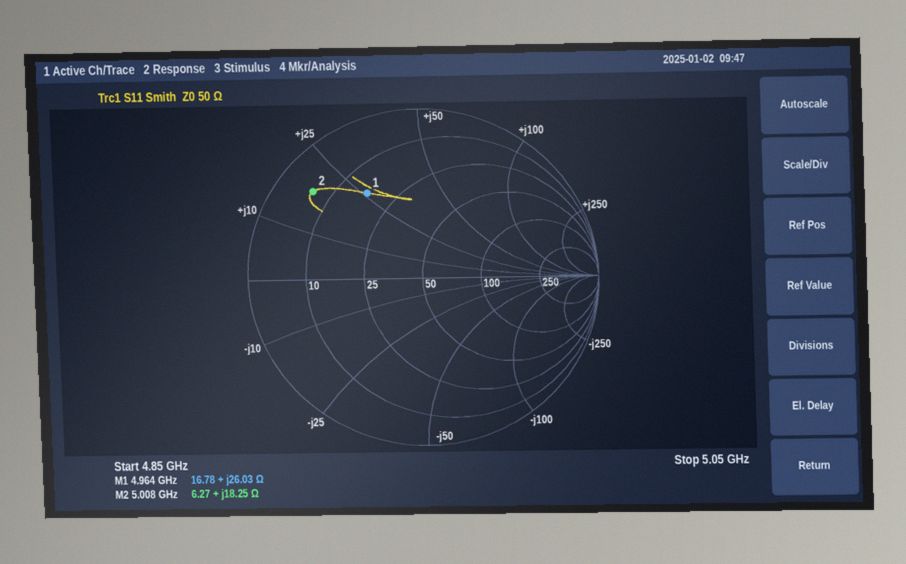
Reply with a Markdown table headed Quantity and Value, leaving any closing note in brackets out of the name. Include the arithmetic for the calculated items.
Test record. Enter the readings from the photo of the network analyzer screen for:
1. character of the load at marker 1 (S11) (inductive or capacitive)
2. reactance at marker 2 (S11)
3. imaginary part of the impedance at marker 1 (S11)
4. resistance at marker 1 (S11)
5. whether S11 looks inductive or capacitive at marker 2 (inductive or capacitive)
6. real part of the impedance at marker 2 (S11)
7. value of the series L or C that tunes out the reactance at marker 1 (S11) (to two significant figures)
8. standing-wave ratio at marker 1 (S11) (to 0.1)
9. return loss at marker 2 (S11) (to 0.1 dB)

| Quantity | Value |
|---|---|
| character of the load at marker 1 (S11) | inductive |
| reactance at marker 2 | +18.25 Ω |
| imaginary part of the impedance at marker 1 | +26.03 Ω |
| resistance at marker 1 | 16.78 Ω |
| whether S11 looks inductive or capacitive at marker 2 | inductive |
| real part of the impedance at marker 2 | 6.27 Ω |
| value of the series L or C that tunes out the reactance at marker 1 (S11) | C = 1/(2π × 4.964 GHz × 26.03 Ω) ≈ 1.2 pF |
| standing-wave ratio at marker 1 (S11) | 3.9 |
| return loss at marker 2 (S11) | 1.9 dB |
